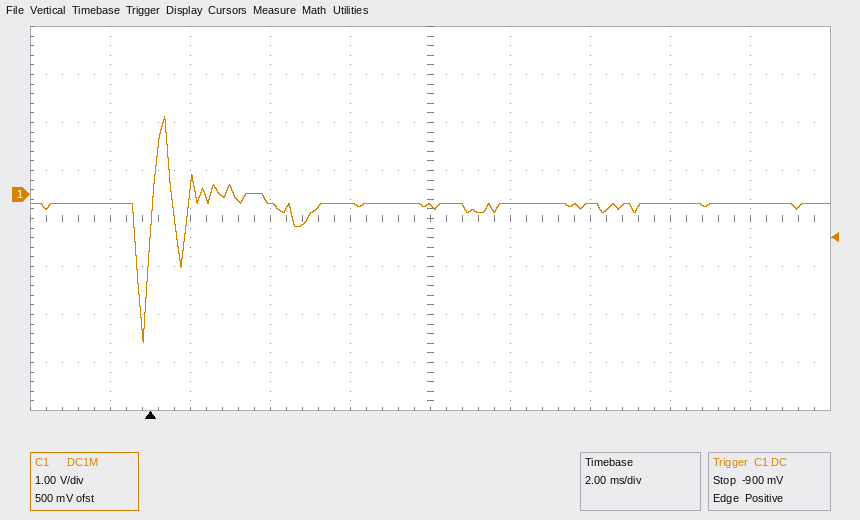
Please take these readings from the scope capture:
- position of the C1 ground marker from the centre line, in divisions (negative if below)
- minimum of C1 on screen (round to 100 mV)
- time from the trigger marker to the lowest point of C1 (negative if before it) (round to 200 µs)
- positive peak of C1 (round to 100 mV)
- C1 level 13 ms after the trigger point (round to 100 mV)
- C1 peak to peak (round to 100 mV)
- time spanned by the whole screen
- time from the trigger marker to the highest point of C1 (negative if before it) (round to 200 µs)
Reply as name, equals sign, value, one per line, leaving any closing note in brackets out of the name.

position of the C1 ground marker from the centre line, in divisions = +0.5 div
minimum of C1 on screen = -3.1 V
time from the trigger marker to the lowest point of C1 (negative if before it) = -200 µs
positive peak of C1 = 1.6 V
C1 level 13 ms after the trigger point = -200 mV
C1 peak to peak = 4.7 V
time spanned by the whole screen = 20 ms
time from the trigger marker to the highest point of C1 (negative if before it) = +400 µs
